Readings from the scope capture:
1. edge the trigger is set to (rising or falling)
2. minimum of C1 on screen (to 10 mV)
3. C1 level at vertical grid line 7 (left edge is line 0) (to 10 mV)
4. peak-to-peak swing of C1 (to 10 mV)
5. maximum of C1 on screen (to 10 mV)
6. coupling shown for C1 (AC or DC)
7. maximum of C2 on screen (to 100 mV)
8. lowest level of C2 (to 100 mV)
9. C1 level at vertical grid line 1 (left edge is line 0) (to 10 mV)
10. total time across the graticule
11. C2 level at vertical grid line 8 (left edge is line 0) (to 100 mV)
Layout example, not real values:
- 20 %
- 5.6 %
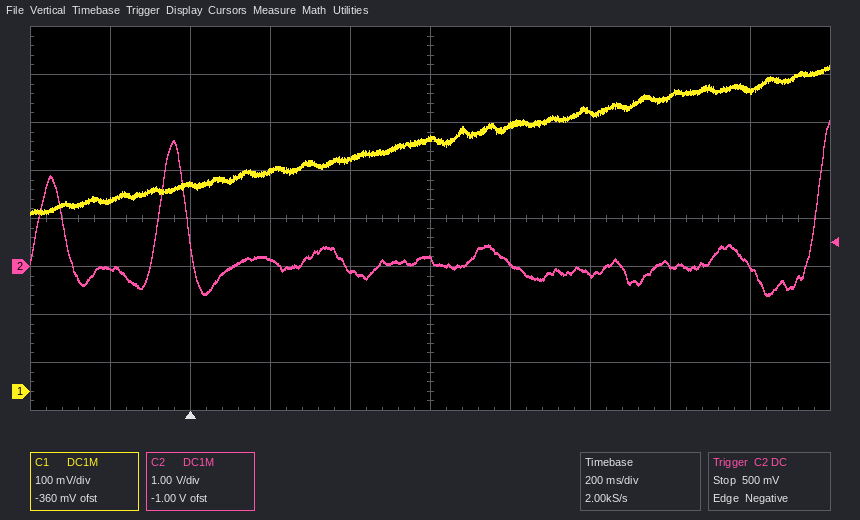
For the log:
- falling
- 370 mV
- 580 mV
- 310 mV
- 680 mV
- DC
- 3.0 V
- -600 mV
- 400 mV
- 2 s
- 0.0 V
